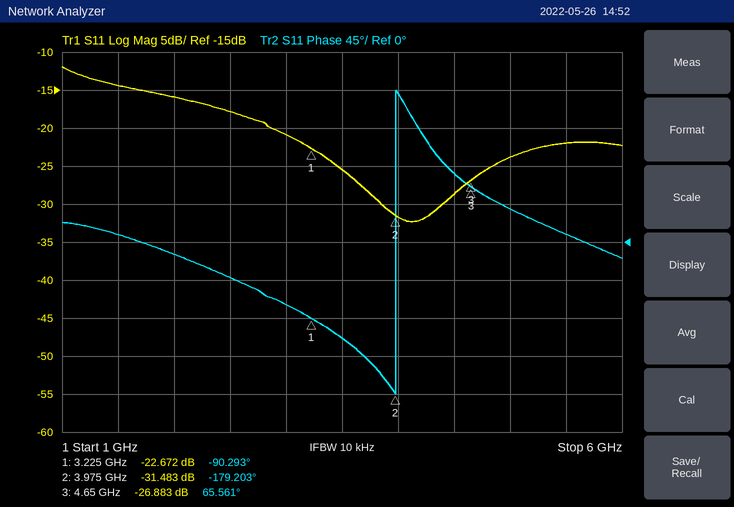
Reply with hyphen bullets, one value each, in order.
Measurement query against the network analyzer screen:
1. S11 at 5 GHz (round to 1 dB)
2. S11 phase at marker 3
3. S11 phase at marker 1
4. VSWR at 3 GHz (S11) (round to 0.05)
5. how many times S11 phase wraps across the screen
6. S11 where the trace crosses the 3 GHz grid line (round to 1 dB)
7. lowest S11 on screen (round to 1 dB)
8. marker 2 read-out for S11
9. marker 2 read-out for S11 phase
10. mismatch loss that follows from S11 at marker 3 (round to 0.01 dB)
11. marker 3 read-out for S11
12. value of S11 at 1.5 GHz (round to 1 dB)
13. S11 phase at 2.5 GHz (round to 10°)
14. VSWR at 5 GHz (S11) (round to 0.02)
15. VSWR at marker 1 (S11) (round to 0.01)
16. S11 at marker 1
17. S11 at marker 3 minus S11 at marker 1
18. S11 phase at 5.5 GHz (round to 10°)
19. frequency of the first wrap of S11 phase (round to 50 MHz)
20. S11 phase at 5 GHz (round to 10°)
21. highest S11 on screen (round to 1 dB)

- -24 dB
- 65.561°
- -90.293°
- 1.20
- 1
- -21 dB
- -32 dB
- -31.483 dB
- -179.203°
- 0.01 dB
- -26.883 dB
- -14 dB
- -40°
- 1.14
- 1.16
- -22.672 dB
- -4.211 dB
- 10°
- 4.00 GHz
- 40°
- -12 dB
